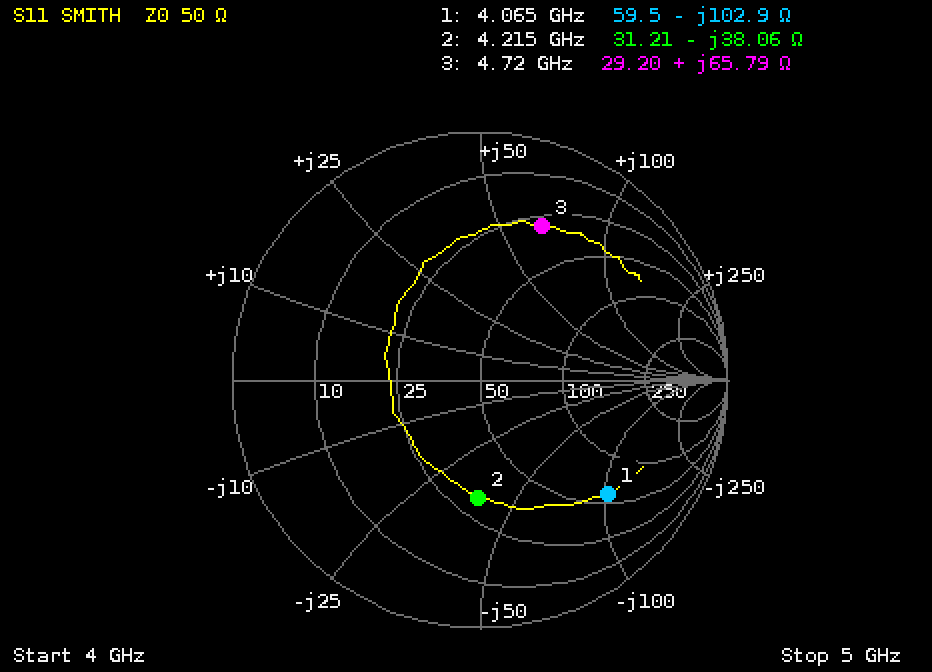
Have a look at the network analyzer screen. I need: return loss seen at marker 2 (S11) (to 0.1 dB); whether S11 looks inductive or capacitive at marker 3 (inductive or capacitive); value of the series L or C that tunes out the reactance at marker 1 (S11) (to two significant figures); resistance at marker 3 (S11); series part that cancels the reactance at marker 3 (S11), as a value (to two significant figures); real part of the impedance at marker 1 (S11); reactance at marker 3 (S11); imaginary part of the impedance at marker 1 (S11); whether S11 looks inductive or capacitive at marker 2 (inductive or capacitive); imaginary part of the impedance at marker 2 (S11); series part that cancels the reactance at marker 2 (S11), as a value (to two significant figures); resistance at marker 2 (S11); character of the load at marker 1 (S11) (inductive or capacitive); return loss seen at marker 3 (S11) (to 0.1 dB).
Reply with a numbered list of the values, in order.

1. 6.5 dB
2. inductive
3. 4.0 nH
4. 29.20 Ω
5. 510 fF
6. 59.5 Ω
7. +65.79 Ω
8. -102.9 Ω
9. capacitive
10. -38.06 Ω
11. 1.4 nH
12. 31.21 Ω
13. capacitive
14. 3.5 dB
